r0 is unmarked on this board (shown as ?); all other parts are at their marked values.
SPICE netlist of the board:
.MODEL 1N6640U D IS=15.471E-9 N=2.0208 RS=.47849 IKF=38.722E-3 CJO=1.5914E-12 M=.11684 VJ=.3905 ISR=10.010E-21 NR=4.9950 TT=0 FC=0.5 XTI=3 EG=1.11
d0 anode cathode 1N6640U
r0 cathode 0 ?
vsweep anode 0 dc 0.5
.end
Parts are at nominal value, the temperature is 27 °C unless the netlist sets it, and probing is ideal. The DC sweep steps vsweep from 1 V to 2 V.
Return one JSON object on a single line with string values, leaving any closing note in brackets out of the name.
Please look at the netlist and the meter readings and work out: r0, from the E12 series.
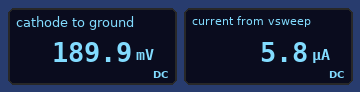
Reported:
{"r0, from the E12 series": "33 kΩ"}
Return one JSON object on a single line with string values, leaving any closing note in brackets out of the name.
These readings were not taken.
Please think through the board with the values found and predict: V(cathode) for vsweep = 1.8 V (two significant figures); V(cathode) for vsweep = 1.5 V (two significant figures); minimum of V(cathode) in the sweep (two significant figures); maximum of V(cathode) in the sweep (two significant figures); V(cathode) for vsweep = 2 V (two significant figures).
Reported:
{"V(cathode) for vsweep = 1.8 V": "1.4 V", "V(cathode) for vsweep = 1.5 V": "1.1 V", "minimum of V(cathode) in the sweep": "630 mV", "maximum of V(cathode) in the sweep": "1.6 V", "V(cathode) for vsweep = 2 V": "1.6 V"}
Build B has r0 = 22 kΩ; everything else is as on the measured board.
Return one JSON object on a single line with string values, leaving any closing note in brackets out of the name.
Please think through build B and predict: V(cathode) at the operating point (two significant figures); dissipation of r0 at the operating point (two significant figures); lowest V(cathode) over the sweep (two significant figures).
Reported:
{"V(cathode) at the operating point": "170 mV", "dissipation of r0 at the operating point": "1.4 µW", "lowest V(cathode) over the sweep": "610 mV"}
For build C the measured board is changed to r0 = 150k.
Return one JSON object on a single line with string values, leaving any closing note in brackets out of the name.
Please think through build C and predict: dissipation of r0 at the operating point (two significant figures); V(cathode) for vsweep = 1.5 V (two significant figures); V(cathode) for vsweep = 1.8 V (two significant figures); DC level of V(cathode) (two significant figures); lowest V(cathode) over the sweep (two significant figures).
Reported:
{"dissipation of r0 at the operating point": "430 nW", "V(cathode) for vsweep = 1.5 V": "1.2 V", "V(cathode) for vsweep = 1.8 V": "1.5 V", "DC level of V(cathode)": "250 mV", "lowest V(cathode) over the sweep": "700 mV"}
